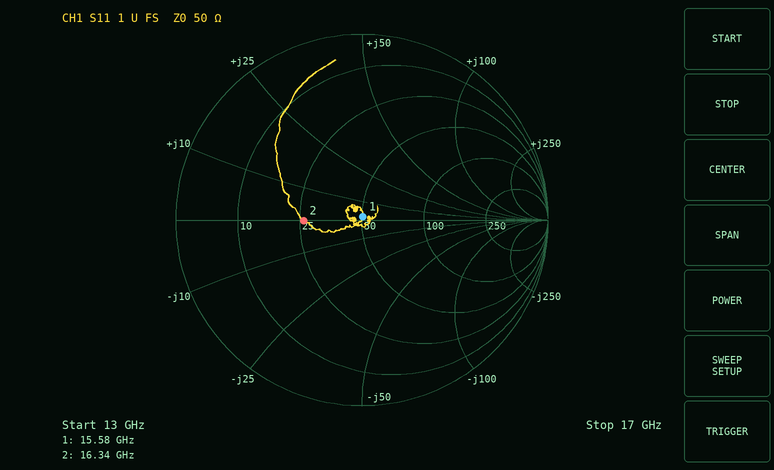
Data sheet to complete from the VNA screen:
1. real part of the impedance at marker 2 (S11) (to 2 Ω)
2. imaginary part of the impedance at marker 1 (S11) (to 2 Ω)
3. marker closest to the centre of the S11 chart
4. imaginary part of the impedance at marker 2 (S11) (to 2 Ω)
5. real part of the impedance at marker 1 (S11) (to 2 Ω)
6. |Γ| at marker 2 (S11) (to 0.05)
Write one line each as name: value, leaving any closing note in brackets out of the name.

real part of the impedance at marker 2 (S11): 26 Ω
imaginary part of the impedance at marker 1 (S11): +2 Ω
marker closest to the centre of the S11 chart: marker 1
imaginary part of the impedance at marker 2 (S11): 0 Ω
real part of the impedance at marker 1 (S11): 50 Ω
|Γ| at marker 2 (S11): 0.30
